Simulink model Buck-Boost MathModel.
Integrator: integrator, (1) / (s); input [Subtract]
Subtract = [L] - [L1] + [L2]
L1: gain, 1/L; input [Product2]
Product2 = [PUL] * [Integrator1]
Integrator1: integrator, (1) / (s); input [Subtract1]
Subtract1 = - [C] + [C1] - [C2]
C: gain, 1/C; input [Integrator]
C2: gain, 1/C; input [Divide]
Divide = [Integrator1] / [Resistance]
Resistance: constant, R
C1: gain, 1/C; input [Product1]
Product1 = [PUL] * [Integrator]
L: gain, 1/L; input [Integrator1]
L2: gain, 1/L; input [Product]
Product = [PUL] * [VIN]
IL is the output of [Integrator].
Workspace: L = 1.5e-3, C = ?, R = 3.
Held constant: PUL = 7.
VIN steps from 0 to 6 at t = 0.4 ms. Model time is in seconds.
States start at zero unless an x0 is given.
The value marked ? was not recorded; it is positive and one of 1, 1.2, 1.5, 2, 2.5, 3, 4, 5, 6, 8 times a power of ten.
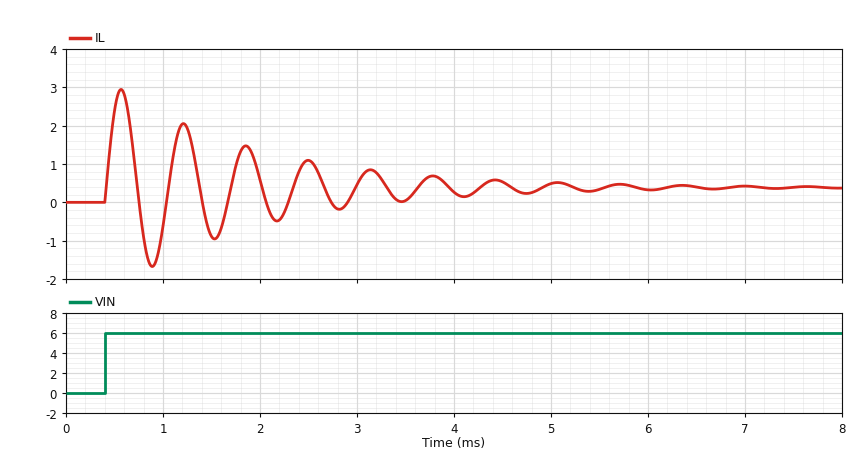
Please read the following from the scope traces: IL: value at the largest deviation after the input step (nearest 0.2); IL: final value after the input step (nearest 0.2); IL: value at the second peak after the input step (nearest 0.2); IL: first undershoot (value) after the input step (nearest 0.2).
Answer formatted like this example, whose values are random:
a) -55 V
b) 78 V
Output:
a) 3.0
b) 0.4
c) 2.0
d) -1.6
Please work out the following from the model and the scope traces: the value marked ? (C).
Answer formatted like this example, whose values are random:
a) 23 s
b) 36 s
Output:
a) 0.00025
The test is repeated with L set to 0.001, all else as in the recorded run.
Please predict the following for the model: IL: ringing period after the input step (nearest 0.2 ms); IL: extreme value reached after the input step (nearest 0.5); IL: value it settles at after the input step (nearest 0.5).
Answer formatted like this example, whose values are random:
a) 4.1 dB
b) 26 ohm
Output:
a) 0.6 ms
b) 3.5
c) 0.5
